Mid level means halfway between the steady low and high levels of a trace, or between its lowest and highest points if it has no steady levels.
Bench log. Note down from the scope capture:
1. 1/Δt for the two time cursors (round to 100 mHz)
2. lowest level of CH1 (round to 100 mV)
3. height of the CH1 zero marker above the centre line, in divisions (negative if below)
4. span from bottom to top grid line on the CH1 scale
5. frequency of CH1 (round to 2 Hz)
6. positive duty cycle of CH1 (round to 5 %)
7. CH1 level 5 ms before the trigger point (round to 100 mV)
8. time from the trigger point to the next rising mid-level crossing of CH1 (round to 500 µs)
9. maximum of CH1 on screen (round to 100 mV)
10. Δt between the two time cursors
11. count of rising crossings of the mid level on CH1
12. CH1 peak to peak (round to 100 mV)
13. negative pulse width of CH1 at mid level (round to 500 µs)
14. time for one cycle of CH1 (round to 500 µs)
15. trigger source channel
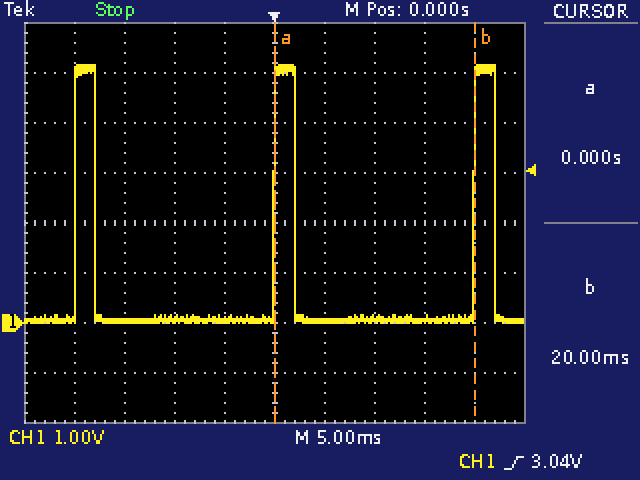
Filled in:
50.0 Hz
0.0 V
-2.0 div
8 V
50 Hz
10 %
100 mV
20.0 ms
5.2 V
20.0 ms
3
5.2 V
18.0 ms
20.0 ms
CH1
